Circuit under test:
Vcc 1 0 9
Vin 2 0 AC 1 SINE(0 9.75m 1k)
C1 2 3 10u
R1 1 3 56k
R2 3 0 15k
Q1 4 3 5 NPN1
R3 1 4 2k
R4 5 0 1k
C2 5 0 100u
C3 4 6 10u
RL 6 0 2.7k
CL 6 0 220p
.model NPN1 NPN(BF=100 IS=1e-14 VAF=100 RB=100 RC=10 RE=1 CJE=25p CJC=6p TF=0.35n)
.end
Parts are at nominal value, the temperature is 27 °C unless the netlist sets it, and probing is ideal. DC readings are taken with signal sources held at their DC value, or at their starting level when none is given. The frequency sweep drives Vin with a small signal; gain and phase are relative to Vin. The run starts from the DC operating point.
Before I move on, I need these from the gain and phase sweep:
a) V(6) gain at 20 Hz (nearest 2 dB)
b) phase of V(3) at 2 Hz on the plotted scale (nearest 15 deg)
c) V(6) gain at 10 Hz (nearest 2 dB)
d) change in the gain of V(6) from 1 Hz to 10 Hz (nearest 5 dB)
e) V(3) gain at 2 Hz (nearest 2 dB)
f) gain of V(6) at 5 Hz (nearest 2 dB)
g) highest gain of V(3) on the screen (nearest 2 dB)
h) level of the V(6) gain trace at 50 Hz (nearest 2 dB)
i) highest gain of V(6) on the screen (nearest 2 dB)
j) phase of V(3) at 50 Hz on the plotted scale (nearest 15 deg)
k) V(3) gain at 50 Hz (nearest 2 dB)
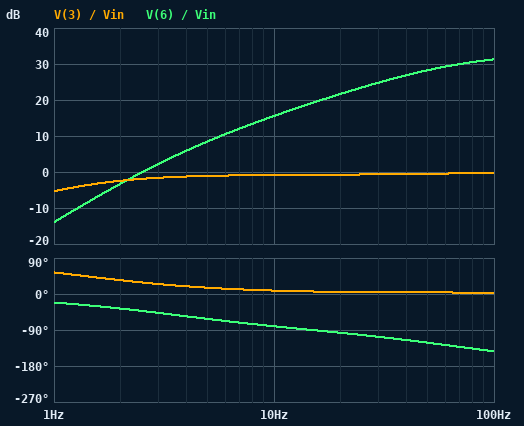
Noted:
22 dB
30 deg
16 dB
30 dB
-2 dB
8 dB
0 dB
28 dB
32 dB
0 deg
0 dB
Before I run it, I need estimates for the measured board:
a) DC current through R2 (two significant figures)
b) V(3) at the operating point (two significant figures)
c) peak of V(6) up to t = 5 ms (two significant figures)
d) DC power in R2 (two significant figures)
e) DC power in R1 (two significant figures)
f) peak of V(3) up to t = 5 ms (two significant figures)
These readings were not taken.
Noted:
120 µA
1.8 V
400 mV
210 µW
930 µW
1.8 V
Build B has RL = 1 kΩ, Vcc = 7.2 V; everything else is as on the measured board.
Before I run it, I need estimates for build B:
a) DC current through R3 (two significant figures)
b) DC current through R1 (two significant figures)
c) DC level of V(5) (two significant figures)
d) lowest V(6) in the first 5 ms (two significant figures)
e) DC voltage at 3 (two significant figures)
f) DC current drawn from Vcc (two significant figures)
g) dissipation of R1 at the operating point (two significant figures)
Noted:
780 µA
100 µA
780 mV
-200 mV
1.4 V
880 µA
590 µW
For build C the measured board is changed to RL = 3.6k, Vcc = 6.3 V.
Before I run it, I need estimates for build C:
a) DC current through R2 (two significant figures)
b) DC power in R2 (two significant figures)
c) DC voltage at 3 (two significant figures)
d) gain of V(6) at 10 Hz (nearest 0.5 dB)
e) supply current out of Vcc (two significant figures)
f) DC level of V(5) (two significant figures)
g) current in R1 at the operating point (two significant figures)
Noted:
84 µA
110 µW
1.3 V
16.5 dB
700 µA
620 mV
90 µA
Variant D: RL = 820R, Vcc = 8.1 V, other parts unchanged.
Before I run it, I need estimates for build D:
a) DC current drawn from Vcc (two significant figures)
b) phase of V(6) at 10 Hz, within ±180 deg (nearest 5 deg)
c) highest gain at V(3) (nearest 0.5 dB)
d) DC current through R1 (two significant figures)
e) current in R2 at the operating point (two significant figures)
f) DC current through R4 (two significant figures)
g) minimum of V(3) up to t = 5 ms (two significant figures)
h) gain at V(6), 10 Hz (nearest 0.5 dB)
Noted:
1.1 mA
-70 deg
0 dB
120 µA
110 µA
950 µA
1.6 V
9.0 dB
